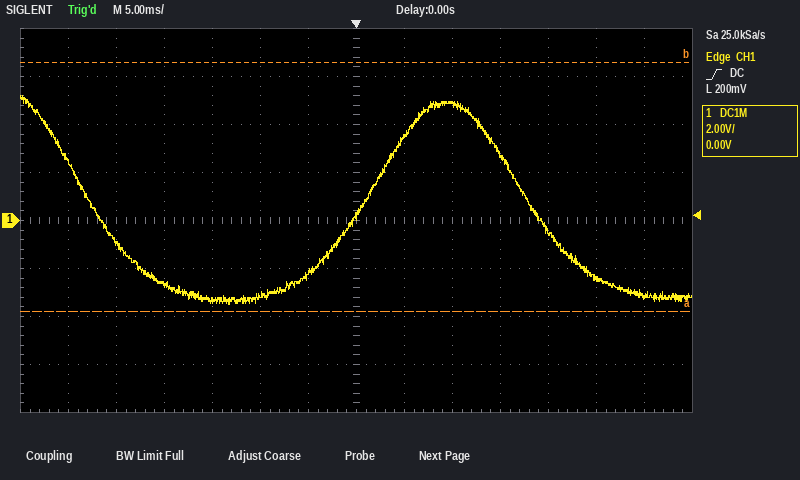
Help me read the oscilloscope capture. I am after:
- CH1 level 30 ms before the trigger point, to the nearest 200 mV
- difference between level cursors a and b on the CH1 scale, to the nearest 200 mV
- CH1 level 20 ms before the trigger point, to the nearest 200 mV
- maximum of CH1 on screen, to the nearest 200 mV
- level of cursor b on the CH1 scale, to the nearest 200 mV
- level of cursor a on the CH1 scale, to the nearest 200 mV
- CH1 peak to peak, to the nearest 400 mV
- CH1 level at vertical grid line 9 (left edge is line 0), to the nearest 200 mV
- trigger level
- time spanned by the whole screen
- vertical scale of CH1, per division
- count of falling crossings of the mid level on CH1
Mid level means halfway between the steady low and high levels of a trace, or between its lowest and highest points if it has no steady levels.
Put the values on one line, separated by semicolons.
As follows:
2.4 V; 10.4 V; -2.6 V; 5.2 V; 6.6 V; -3.8 V; 8.8 V; 4.8 V; 200 mV; 70 ms; 2 V; 2
